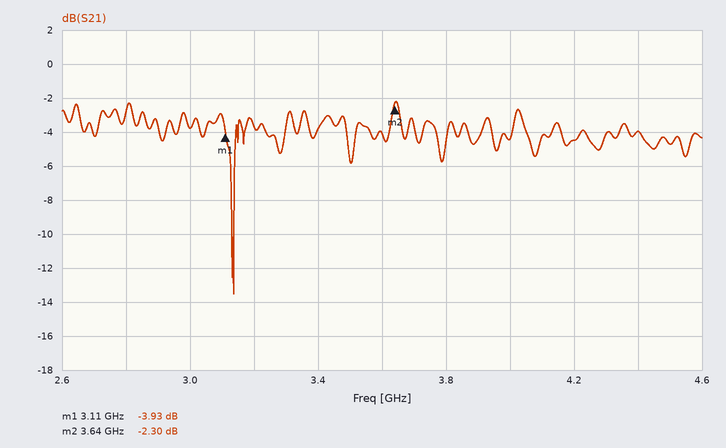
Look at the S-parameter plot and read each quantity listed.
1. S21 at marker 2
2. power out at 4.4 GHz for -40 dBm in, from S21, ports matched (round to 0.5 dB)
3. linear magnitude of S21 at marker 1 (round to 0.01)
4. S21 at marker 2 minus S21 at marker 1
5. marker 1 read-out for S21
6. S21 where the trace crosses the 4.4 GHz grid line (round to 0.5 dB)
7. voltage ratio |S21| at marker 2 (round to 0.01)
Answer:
-2.30 dB
-44.0 dBm
0.64
1.63 dB
-3.93 dB
-4.0 dB
0.77
